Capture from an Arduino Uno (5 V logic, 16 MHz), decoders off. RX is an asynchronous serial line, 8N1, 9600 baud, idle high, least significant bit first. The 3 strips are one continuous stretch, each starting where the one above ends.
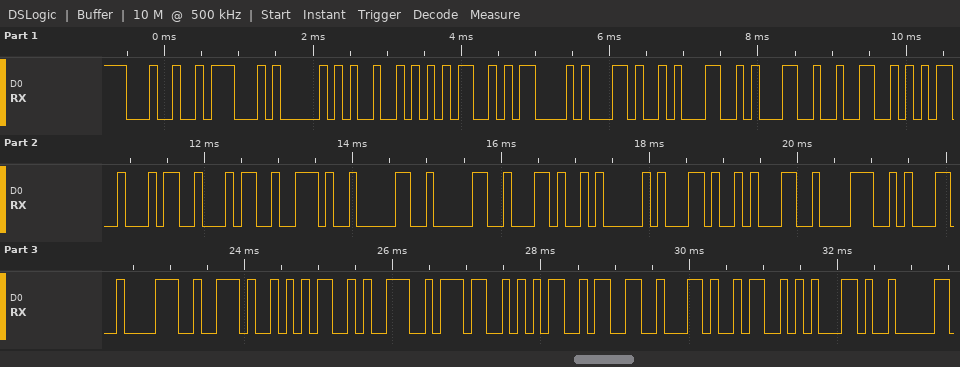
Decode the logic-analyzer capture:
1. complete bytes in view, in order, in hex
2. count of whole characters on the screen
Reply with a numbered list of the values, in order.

1. 0x24 0x47 0x50 0x52 0x4D 0x43 0x2C 0x31 0x31 0x32 0x35 0x34 0x34 0x2E 0x30 0x30 0x2C 0x41 0x2C 0x31 0x38 0x31 0x38 0x2E 0x35 0x39 0x37 0x35 0x33 0x2C 0x53 0x2C
2. 32
